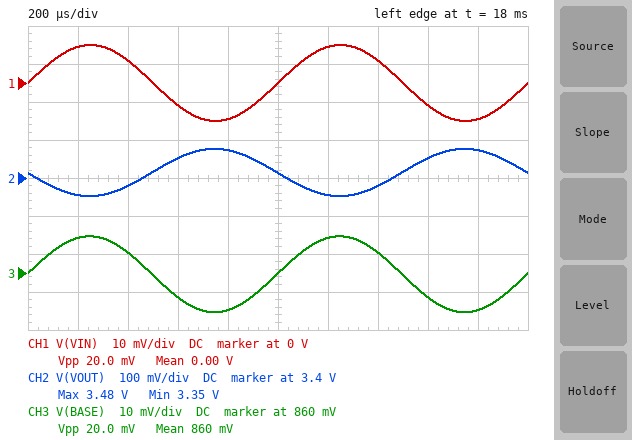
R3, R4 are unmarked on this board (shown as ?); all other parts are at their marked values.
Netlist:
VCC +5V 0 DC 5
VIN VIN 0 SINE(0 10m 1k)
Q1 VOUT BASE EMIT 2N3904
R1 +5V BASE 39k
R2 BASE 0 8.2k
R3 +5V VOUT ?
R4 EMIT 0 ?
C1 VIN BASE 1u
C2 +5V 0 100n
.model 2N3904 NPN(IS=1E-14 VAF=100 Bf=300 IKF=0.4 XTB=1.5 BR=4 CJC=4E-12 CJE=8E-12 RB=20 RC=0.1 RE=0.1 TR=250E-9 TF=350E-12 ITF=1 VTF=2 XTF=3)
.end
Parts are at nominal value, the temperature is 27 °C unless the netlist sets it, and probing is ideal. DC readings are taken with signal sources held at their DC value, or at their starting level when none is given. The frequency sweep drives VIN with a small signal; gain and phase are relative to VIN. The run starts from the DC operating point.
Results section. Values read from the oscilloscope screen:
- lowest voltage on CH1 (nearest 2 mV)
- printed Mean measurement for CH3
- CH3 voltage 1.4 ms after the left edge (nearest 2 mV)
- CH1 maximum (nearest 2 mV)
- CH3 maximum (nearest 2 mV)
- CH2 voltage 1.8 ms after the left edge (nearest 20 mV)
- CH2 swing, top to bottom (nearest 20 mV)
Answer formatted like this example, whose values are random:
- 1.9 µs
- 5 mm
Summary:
- -10 mV
- 860 mV
- 866 mV
- 10 mV
- 870 mV
- 3.48 V
- 120 mV
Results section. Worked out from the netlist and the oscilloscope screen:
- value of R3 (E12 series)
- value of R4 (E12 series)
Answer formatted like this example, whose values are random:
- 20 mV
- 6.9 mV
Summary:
- 3.9 kΩ
- 560 Ω
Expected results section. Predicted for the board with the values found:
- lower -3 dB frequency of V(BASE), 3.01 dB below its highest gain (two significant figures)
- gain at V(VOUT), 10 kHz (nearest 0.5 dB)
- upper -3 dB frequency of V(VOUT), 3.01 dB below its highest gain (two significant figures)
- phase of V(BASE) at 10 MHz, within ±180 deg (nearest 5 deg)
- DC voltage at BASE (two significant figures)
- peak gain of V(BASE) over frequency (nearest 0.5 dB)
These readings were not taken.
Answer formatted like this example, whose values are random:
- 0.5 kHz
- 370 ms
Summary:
- 24 Hz
- 16.0 dB
- 17 MHz
- 0 deg
- 860 mV
- 0 dB
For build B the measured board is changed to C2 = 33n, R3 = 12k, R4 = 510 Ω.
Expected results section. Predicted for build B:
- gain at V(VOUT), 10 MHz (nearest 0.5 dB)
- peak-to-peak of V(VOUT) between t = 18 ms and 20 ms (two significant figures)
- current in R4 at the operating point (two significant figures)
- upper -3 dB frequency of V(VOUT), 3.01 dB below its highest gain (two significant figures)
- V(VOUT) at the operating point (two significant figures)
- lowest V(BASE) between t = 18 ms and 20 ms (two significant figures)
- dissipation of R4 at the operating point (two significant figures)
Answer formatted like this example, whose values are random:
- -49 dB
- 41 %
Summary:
- 0 dB
- 210 mV
- 400 µA
- 320 kHz
- 290 mV
- 820 mV
- 81 µW
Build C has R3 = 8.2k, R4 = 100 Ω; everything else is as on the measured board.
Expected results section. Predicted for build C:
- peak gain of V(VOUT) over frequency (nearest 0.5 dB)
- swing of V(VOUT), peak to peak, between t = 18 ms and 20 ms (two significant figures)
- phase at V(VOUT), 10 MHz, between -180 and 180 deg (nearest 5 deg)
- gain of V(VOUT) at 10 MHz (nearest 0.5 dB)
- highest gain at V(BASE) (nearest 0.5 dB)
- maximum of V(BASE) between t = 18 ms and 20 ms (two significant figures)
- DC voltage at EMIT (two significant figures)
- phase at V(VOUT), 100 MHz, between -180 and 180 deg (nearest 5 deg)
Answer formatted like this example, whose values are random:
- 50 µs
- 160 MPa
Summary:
- 9.0 dB
- 180 mV
- 10 deg
- -1.0 dB
- 0 dB
- 720 mV
- 62 mV
- 0 deg
